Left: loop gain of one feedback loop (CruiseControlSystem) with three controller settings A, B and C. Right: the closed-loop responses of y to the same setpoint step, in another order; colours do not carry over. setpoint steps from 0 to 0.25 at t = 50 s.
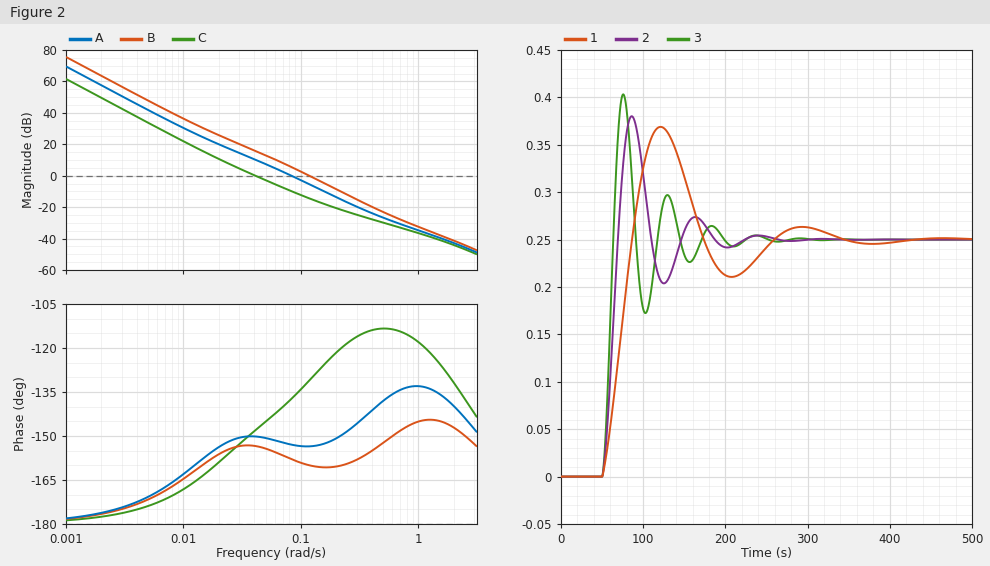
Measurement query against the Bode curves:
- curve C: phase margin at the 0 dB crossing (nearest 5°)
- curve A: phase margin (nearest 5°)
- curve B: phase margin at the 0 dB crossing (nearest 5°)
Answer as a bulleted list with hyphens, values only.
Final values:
- 30°
- 25°
- 20°
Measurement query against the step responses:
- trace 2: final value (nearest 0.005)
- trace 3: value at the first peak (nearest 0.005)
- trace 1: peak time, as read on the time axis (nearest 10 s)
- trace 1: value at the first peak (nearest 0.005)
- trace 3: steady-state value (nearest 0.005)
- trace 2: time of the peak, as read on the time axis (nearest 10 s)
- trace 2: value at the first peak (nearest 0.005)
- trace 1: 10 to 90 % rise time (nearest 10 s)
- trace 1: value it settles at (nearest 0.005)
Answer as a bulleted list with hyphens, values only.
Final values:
- 0.250
- 0.405
- 120 s
- 0.370
- 0.250
- 90 s
- 0.380
- 30 s
- 0.250
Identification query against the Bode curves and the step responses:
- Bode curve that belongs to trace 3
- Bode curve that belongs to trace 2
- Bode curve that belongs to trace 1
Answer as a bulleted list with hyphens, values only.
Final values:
- B
- A
- C
